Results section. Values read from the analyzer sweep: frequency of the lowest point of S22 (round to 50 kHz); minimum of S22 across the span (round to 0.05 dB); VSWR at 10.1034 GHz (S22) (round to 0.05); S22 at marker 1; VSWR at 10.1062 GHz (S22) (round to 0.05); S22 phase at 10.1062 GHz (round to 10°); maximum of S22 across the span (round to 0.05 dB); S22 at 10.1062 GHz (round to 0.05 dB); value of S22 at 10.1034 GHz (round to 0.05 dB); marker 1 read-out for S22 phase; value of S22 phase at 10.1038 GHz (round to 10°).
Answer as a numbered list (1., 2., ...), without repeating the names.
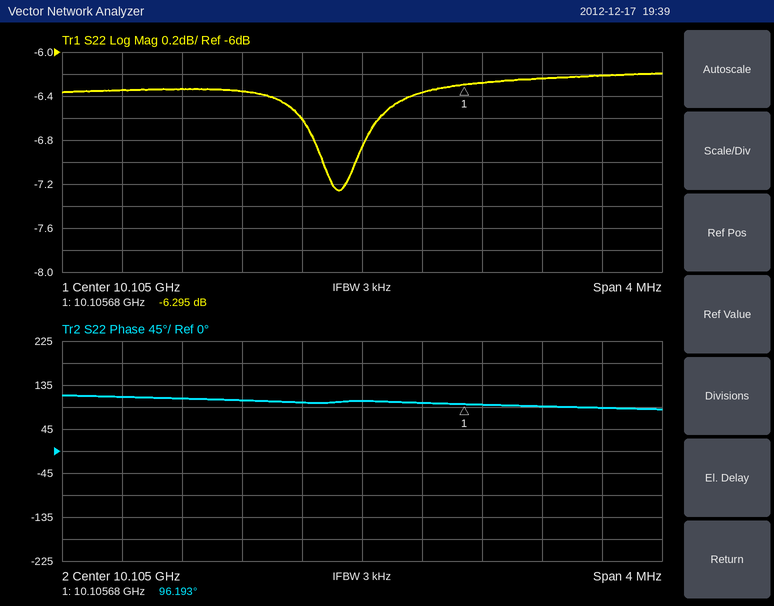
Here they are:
1. 10.10485 GHz
2. -7.25 dB
3. 2.85
4. -6.295 dB
5. 2.90
6. 90°
7. -6.20 dB
8. -6.25 dB
9. -6.35 dB
10. 96.193°
11. 110°
